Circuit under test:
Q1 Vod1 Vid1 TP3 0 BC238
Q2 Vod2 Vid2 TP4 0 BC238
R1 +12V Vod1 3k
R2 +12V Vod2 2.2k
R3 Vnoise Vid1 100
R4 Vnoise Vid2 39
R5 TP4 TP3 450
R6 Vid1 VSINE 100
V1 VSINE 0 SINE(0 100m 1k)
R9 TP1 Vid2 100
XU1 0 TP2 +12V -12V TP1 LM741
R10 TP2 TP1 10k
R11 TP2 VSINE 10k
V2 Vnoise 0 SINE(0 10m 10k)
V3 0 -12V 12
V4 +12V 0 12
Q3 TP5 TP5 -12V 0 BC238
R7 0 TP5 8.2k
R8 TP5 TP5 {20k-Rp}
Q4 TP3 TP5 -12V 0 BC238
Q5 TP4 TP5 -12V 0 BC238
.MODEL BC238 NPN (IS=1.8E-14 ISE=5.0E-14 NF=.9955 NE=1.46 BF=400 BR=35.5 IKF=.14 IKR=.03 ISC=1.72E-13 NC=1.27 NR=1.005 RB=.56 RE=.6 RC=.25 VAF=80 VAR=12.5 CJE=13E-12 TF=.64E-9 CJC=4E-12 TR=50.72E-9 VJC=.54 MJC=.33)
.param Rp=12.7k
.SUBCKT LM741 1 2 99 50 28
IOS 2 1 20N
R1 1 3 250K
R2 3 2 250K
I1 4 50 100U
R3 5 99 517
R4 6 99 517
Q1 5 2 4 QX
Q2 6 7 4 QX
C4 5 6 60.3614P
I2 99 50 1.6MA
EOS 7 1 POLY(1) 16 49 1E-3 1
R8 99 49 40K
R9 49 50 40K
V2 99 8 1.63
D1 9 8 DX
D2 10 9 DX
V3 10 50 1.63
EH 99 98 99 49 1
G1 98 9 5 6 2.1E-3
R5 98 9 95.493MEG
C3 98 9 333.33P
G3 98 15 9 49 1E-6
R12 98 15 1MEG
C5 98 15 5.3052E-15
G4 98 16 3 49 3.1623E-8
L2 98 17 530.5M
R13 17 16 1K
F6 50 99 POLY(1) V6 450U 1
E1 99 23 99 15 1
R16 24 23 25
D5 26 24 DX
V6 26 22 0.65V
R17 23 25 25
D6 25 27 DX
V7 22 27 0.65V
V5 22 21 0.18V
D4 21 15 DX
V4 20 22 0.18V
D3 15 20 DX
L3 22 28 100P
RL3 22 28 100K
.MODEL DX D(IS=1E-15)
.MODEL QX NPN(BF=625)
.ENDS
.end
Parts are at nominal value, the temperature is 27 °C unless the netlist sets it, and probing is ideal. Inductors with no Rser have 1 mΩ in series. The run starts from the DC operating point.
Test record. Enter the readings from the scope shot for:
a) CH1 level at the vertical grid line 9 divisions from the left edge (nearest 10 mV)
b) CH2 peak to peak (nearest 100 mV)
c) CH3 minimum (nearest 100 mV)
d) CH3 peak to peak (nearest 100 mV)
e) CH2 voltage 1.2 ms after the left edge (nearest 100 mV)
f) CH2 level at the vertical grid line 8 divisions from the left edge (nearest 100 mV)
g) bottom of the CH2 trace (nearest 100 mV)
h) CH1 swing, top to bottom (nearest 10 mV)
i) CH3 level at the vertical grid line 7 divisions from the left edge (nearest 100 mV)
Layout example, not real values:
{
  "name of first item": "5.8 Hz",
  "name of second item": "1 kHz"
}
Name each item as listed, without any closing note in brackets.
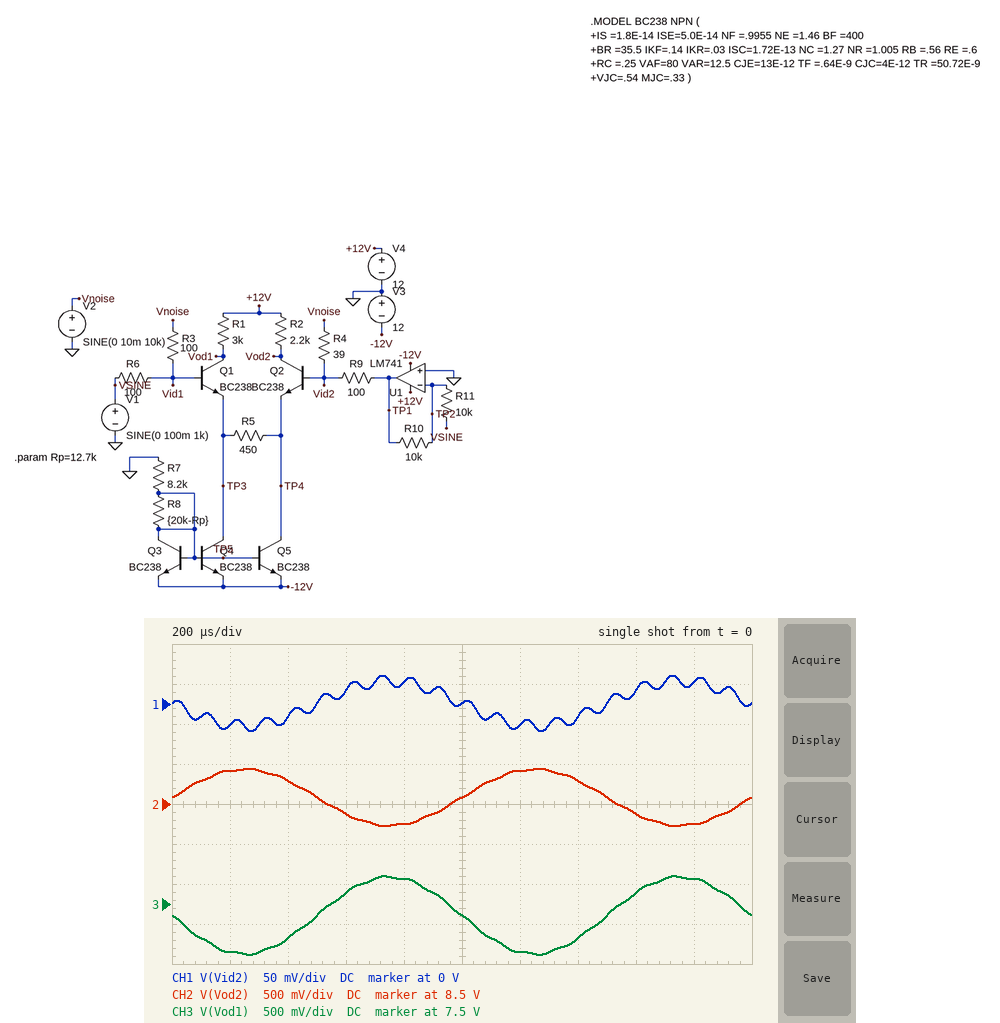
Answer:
{
  "CH1 level at the vertical grid line 9 divisions from the left edge": "30 mV",
  "CH2 peak to peak": "700 mV",
  "CH3 minimum": "6.9 V",
  "CH3 peak to peak": "1.0 V",
  "CH2 voltage 1.2 ms after the left edge": "8.9 V",
  "CH2 level at the vertical grid line 8 divisions from the left edge": "8.4 V",
  "bottom of the CH2 trace": "8.2 V",
  "CH1 swing, top to bottom": "70 mV",
  "CH3 level at the vertical grid line 7 divisions from the left edge": "7.1 V"
}
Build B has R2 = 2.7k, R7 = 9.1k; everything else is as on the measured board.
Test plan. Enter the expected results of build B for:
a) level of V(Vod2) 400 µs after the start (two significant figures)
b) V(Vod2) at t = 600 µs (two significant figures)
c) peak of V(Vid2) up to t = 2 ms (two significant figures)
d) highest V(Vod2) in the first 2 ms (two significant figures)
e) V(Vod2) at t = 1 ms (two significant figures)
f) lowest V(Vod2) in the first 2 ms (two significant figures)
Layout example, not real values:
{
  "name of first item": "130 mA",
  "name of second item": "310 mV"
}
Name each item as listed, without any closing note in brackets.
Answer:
{
  "level of V(Vod2) 400 µs after the start": "8.5 V",
  "V(Vod2) at t = 600 µs": "8.0 V",
  "peak of V(Vid2) up to t = 2 ms": "36 mV",
  "highest V(Vod2) in the first 2 ms": "8.7 V",
  "V(Vod2) at t = 1 ms": "8.2 V",
  "lowest V(Vod2) in the first 2 ms": "7.8 V"
}
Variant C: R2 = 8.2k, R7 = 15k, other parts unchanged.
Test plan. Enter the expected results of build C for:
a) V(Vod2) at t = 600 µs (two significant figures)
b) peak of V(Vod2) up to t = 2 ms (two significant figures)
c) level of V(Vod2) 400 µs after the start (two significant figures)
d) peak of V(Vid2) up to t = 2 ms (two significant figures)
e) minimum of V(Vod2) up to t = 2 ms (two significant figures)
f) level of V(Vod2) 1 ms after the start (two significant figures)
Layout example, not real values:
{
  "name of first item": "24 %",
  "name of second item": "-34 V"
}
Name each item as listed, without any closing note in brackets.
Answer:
{
  "V(Vod2) at t = 600 µs": "4.3 V",
  "peak of V(Vod2) up to t = 2 ms": "6.3 V",
  "level of V(Vod2) 400 µs after the start": "5.8 V",
  "peak of V(Vid2) up to t = 2 ms": "36 mV",
  "minimum of V(Vod2) up to t = 2 ms": "3.8 V",
  "level of V(Vod2) 1 ms after the start": "5.0 V"
}
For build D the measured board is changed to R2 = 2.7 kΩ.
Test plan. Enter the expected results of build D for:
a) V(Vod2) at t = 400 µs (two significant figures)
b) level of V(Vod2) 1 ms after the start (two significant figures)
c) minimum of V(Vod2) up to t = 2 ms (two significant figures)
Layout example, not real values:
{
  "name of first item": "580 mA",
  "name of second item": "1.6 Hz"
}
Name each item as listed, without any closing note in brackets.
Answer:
{
  "V(Vod2) at t = 400 µs": "8.1 V",
  "level of V(Vod2) 1 ms after the start": "7.8 V",
  "minimum of V(Vod2) up to t = 2 ms": "7.4 V"
}
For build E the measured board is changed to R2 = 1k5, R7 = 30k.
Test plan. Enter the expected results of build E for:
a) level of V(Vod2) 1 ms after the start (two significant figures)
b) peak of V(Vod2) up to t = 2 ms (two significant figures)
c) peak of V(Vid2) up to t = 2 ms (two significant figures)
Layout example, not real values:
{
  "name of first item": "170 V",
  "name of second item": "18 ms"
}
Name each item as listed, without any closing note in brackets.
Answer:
{
  "level of V(Vod2) 1 ms after the start": "11 V",
  "peak of V(Vod2) up to t = 2 ms": "12 V",
  "peak of V(Vid2) up to t = 2 ms": "36 mV"
}
